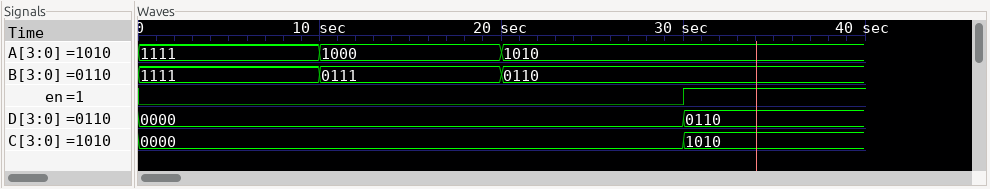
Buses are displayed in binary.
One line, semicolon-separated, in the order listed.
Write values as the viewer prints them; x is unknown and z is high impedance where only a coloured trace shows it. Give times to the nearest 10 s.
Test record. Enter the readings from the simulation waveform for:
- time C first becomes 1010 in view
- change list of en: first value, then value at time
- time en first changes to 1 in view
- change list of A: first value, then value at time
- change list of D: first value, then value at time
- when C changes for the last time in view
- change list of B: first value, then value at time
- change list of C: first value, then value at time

30 s; 0, 1 at 30 s; 30 s; 1111, 1000 at 10 s, 1010 at 20 s; 0000, 0110 at 30 s; 30 s; 1111, 0111 at 10 s, 0110 at 20 s; 0000, 1010 at 30 s
